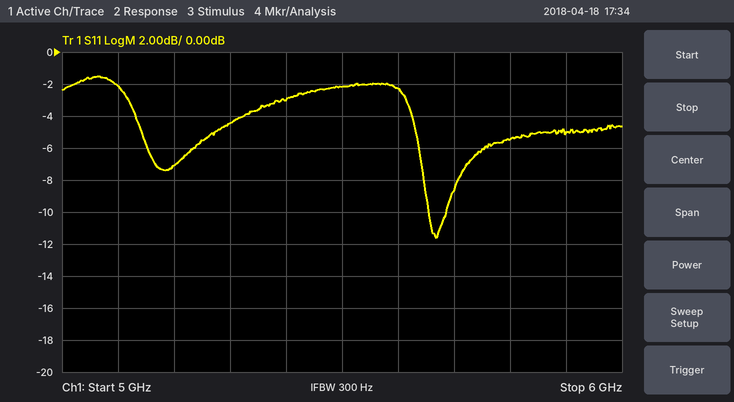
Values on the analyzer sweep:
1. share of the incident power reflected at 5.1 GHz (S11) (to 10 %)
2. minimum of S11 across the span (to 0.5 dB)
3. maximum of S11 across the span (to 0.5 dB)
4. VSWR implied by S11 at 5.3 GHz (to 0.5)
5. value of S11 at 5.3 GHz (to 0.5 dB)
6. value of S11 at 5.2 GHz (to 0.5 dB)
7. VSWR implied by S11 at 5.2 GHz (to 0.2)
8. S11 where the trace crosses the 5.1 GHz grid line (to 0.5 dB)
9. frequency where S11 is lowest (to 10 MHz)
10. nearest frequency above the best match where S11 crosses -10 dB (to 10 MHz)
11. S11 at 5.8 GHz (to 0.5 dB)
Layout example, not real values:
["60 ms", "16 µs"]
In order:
["60 %", "-11.5 dB", "-1.5 dB", "4.0", "-4.5 dB", "-7.0 dB", "2.6", "-2.0 dB", "5.67 GHz", "5.69 GHz", "-5.5 dB"]
